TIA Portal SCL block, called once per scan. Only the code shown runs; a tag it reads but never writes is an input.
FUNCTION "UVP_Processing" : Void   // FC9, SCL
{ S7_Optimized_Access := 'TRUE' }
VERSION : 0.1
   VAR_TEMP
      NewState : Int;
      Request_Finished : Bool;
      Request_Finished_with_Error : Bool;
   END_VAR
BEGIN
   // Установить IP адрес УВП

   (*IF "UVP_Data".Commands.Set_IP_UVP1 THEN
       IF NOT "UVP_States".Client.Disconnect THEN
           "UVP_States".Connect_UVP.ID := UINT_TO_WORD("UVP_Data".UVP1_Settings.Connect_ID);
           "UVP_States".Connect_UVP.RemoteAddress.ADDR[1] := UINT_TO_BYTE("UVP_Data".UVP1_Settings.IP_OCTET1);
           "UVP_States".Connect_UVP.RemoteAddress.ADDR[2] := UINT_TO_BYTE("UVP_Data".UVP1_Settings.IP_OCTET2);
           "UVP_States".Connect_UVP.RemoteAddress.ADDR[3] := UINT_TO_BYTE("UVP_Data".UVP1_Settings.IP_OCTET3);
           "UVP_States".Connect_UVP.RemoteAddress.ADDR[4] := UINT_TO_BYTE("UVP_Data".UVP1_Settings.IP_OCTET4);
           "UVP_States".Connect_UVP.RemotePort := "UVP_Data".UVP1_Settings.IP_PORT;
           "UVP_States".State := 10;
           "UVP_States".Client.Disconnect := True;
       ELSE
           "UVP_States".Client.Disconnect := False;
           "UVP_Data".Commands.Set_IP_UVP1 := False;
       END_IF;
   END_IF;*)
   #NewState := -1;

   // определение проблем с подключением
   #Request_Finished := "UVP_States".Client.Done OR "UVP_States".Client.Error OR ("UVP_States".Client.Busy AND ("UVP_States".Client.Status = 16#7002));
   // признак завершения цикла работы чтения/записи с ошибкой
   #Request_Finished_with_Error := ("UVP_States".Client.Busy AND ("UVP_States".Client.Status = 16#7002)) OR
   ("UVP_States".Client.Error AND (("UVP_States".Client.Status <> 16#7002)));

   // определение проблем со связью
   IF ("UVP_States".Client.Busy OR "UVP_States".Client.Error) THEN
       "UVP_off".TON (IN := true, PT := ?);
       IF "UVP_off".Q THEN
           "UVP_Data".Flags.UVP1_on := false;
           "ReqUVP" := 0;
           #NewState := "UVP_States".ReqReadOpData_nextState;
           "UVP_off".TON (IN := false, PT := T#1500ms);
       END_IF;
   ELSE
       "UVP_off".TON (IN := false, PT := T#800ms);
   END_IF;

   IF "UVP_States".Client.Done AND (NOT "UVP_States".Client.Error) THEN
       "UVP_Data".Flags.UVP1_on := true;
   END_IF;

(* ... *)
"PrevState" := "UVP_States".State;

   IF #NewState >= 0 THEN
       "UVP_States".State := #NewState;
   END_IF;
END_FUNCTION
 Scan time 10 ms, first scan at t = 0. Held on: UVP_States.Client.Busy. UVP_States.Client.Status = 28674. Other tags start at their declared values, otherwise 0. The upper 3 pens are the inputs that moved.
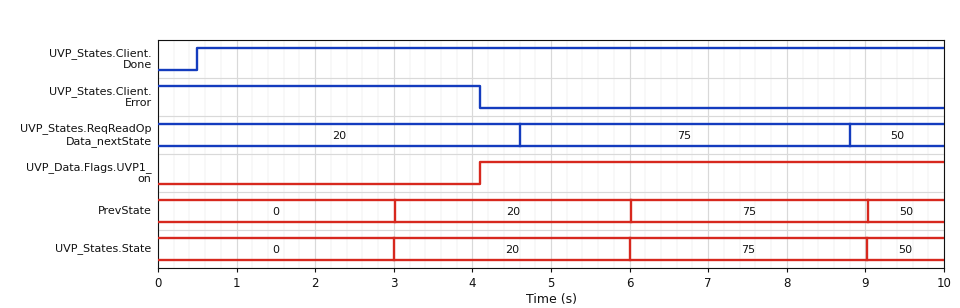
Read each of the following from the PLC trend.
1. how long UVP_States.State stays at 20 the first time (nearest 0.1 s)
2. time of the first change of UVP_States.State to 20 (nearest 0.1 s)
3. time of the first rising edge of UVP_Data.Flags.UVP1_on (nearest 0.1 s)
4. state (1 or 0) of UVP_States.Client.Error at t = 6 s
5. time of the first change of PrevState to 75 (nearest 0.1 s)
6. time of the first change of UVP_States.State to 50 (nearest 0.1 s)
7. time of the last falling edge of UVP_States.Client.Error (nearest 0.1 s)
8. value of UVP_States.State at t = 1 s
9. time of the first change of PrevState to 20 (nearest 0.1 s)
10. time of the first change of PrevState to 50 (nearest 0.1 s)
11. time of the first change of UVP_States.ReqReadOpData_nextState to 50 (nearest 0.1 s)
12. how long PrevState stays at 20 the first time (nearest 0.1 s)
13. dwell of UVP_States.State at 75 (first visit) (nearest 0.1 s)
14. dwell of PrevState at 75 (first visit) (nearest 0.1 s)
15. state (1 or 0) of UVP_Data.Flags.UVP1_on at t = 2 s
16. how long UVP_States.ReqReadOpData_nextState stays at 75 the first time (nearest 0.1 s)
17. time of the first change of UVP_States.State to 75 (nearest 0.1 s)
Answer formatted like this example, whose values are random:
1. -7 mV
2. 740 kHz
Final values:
1. 3.0 s
2. 3.0 s
3. 4.1 s
4. 0
5. 6.0 s
6. 9.0 s
7. 4.1 s
8. 0
9. 3.0 s
10. 9.0 s
11. 8.8 s
12. 3.0 s
13. 3.0 s
14. 3.0 s
15. 0
16. 4.2 s
17. 6.0 s
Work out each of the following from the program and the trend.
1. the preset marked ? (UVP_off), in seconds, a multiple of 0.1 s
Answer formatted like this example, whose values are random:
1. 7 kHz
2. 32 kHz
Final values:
1. 3.0 s
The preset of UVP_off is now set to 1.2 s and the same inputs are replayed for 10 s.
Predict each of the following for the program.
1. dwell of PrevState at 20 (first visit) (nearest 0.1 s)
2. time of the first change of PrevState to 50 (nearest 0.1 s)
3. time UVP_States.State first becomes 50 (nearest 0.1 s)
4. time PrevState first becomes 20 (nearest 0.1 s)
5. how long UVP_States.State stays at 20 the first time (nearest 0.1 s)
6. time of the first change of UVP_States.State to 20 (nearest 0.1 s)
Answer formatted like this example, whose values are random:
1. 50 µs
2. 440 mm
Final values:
1. 3.6 s
2. 9.7 s
3. 9.7 s
4. 1.2 s
5. 3.6 s
6. 1.2 s
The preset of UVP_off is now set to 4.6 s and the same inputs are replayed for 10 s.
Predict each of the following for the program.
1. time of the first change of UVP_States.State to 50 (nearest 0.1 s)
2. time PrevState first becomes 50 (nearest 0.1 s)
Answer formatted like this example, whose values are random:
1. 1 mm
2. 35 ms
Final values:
1. 9.2 s
2. 9.2 s
